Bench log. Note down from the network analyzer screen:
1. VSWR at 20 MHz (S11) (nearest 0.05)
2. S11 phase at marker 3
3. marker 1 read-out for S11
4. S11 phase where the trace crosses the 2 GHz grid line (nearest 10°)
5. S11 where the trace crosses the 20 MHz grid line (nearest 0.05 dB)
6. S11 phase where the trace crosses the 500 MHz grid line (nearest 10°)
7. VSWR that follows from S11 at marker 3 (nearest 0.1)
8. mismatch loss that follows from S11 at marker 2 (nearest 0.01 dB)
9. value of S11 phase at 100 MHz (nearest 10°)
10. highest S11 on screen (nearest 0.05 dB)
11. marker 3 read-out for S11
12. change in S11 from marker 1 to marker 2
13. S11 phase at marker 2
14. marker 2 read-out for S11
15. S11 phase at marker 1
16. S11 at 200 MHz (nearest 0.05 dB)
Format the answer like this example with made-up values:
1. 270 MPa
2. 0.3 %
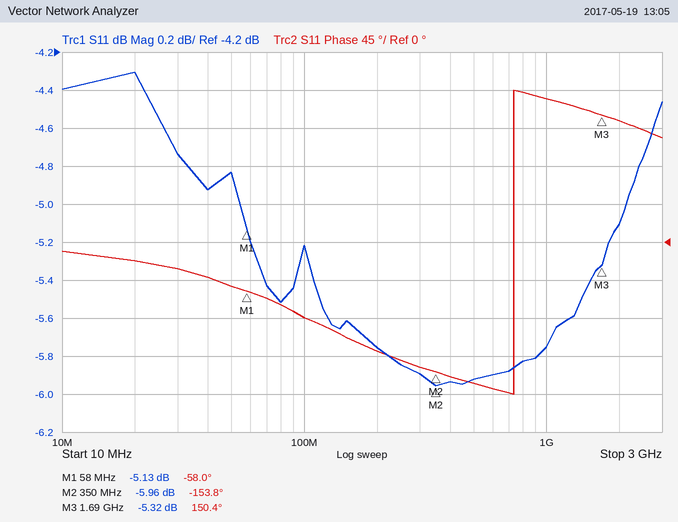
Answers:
1. 4.10
2. 150.4°
3. -5.13 dB
4. 140°
5. -4.30 dB
6. -170°
7. 3.4
8. 1.27 dB
9. -90°
10. -4.30 dB
11. -5.32 dB
12. -0.83 dB
13. -153.8°
14. -5.96 dB
15. -58.0°
16. -5.75 dB
